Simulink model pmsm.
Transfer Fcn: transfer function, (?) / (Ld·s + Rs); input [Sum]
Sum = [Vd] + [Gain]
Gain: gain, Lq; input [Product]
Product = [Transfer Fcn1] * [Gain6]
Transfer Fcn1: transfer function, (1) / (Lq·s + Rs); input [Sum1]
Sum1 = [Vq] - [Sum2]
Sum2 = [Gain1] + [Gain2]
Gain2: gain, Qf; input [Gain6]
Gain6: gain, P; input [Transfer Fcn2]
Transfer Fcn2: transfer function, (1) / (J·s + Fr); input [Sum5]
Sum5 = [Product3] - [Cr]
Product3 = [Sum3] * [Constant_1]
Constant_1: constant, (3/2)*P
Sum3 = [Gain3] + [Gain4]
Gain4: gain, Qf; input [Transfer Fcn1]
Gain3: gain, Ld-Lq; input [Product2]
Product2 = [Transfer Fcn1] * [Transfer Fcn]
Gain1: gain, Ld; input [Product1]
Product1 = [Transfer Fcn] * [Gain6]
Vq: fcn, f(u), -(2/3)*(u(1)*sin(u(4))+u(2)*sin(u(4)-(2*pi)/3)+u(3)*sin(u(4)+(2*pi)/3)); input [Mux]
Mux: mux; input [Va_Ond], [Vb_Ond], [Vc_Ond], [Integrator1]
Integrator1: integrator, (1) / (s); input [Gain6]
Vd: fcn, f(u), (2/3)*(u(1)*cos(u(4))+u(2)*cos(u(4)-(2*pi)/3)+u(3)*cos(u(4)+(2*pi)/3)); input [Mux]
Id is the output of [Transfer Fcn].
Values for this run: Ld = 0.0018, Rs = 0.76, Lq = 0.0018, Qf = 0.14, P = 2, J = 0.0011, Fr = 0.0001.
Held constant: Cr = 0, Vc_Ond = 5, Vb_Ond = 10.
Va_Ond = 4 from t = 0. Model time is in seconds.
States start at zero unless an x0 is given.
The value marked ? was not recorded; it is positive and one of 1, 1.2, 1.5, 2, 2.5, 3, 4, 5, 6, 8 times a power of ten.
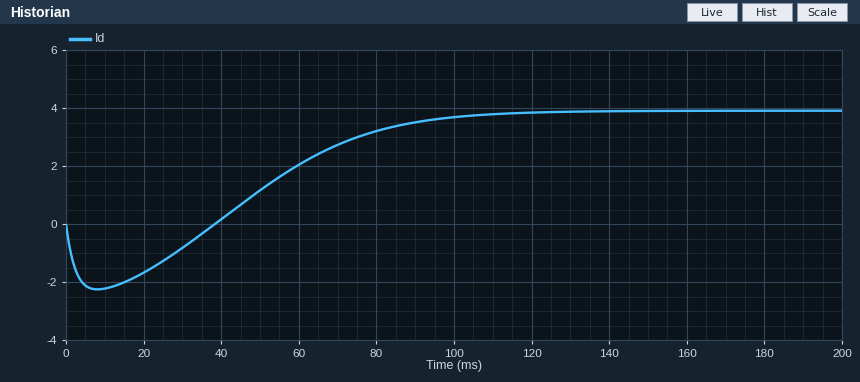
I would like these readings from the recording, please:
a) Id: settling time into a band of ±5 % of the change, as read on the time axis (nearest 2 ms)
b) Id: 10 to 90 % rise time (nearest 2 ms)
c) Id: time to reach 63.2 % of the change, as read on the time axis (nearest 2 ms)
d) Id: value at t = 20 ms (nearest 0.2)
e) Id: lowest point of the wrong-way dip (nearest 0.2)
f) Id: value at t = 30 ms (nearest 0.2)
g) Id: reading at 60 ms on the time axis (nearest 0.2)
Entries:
102 ms
48 ms
66 ms
-1.6
-2.2
-0.8
2.0
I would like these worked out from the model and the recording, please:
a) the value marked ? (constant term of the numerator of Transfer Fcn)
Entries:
0.8
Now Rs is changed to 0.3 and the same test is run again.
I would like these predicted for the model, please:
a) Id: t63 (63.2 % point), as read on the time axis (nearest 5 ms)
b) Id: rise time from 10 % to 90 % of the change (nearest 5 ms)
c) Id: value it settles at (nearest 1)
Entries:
65 ms
55 ms
10
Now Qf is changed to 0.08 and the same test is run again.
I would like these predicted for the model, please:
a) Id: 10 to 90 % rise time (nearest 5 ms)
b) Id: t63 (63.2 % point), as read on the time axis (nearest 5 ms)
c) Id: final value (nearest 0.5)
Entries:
30 ms
55 ms
4.0
